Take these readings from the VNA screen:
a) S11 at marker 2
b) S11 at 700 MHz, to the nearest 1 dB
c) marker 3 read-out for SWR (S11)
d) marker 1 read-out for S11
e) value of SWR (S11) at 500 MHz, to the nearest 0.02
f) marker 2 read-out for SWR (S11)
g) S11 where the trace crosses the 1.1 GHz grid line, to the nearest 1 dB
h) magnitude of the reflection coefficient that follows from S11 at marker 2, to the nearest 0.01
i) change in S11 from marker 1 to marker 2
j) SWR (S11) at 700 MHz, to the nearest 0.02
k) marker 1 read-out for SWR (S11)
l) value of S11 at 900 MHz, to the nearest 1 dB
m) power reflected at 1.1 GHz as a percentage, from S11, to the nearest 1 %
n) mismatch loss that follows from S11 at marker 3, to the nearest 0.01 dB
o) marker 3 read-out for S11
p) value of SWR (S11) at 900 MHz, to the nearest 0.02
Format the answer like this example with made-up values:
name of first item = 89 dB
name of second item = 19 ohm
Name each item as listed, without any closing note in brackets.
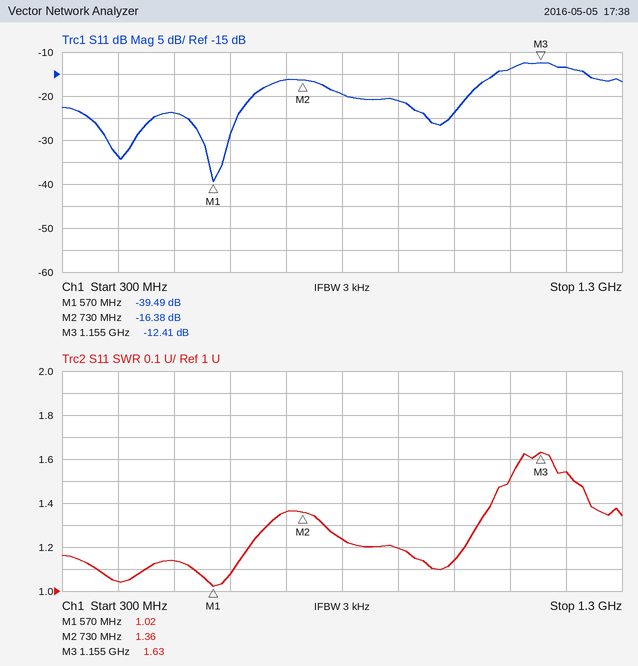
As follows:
S11 at marker 2 = -16.38 dB
S11 at 700 MHz, to the nearest 1 dB = -16 dB
marker 3 read-out for SWR = 1.63
marker 1 read-out for S11 = -39.49 dB
value of SWR (S11) at 500 MHz, to the nearest 0.02 = 1.14
marker 2 read-out for SWR = 1.36
S11 where the trace crosses the 1.1 GHz grid line, to the nearest 1 dB = -14 dB
magnitude of the reflection coefficient that follows from S11 at marker 2, to the nearest 0.01 = 0.15
change in S11 from marker 1 to marker 2 = 23.11 dB
SWR (S11) at 700 MHz, to the nearest 0.02 = 1.36
marker 1 read-out for SWR = 1.02
value of S11 at 900 MHz, to the nearest 1 dB = -21 dB
power reflected at 1.1 GHz as a percentage, from S11, to the nearest 1 % = 4 %
mismatch loss that follows from S11 at marker 3, to the nearest 0.01 dB = 0.26 dB
marker 3 read-out for S11 = -12.41 dB
value of SWR (S11) at 900 MHz, to the nearest 0.02 = 1.20
